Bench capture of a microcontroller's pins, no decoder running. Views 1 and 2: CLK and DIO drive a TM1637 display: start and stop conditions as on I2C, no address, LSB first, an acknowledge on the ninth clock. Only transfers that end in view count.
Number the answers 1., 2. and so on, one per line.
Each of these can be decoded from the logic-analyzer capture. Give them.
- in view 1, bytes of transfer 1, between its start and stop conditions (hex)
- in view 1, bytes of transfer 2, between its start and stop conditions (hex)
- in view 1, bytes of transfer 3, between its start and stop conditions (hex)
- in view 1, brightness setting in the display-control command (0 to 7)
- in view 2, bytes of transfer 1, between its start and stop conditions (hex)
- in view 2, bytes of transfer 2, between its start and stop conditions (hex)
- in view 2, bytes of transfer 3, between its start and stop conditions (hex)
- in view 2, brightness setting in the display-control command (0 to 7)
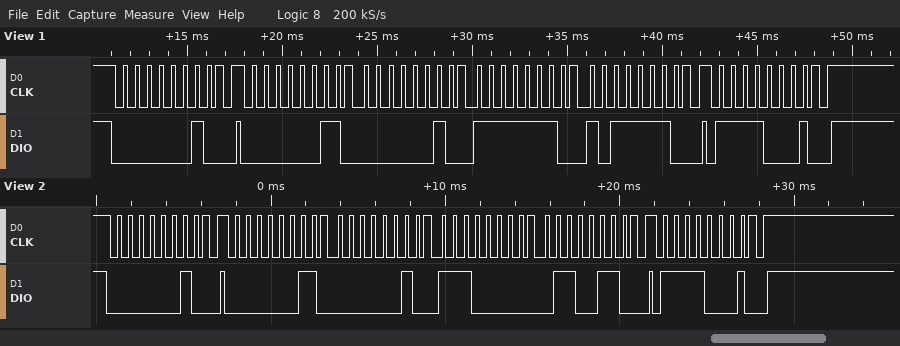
1. 40
2. C0 40 7F 7D
3. 8F
4. 7
5. 40
6. C0 40 07 66
7. 8F
8. 7
